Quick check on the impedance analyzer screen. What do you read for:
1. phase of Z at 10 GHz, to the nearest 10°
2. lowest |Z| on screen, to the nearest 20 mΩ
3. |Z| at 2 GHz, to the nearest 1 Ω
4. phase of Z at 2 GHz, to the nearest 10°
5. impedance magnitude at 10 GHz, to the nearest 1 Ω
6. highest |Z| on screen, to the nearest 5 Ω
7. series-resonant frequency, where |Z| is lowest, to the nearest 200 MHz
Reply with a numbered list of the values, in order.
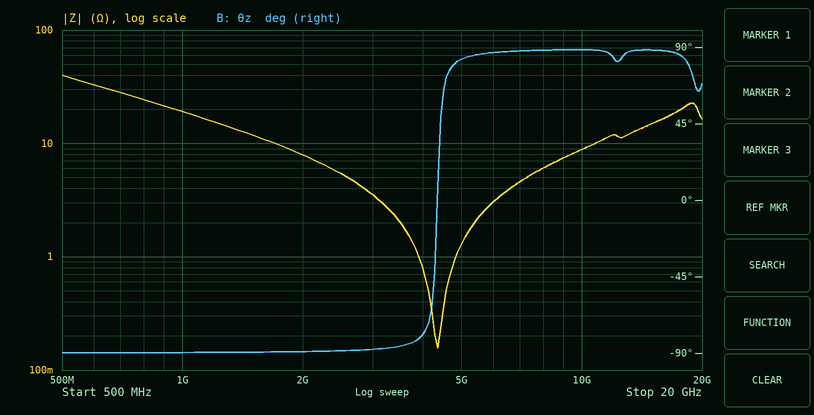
1. 90°
2. 160 mΩ
3. 8 Ω
4. -90°
5. 9 Ω
6. 40 Ω
7. 4.4 GHz
